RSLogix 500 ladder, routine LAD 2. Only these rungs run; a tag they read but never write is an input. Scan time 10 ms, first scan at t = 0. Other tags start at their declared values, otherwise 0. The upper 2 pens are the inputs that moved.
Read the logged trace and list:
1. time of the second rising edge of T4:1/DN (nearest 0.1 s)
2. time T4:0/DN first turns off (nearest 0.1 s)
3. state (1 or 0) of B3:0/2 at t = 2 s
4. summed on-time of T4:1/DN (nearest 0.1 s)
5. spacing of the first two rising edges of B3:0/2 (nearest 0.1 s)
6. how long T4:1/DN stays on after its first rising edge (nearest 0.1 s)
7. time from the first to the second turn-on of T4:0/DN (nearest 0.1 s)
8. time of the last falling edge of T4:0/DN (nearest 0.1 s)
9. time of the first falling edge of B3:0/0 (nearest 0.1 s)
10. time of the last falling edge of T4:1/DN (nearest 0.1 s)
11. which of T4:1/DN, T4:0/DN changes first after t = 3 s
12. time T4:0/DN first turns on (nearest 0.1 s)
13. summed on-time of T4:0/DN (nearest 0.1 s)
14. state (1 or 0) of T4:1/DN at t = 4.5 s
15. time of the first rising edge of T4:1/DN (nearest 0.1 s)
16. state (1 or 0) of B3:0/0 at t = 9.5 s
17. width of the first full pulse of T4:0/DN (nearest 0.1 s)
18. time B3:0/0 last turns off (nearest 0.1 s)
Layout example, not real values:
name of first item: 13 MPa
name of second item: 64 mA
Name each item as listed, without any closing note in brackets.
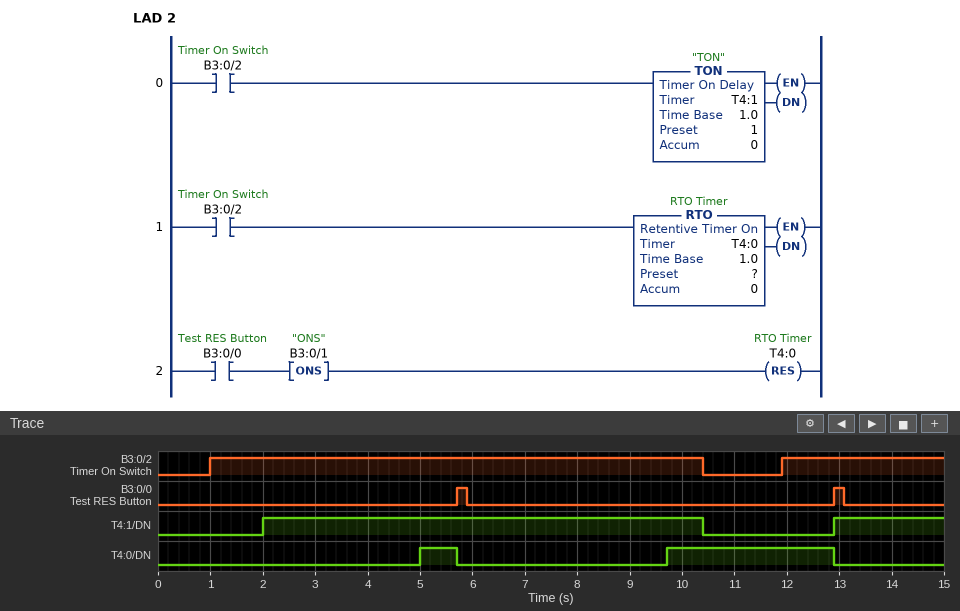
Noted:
time of the second rising edge of T4:1/DN: 12.9 s
time T4:0/DN first turns off: 5.7 s
state (1 or 0) of B3:0/2 at t = 2 s: 1
summed on-time of T4:1/DN: 10.5 s
spacing of the first two rising edges of B3:0/2: 10.9 s
how long T4:1/DN stays on after its first rising edge: 8.4 s
time from the first to the second turn-on of T4:0/DN: 4.7 s
time of the last falling edge of T4:0/DN: 12.9 s
time of the first falling edge of B3:0/0: 5.9 s
time of the last falling edge of T4:1/DN: 10.4 s
which of T4:1/DN, T4:0/DN changes first after t = 3 s: T4:0/DN
time T4:0/DN first turns on: 5.0 s
summed on-time of T4:0/DN: 3.9 s
state (1 or 0) of T4:1/DN at t = 4.5 s: 1
time of the first rising edge of T4:1/DN: 2.0 s
state (1 or 0) of B3:0/0 at t = 9.5 s: 0
width of the first full pulse of T4:0/DN: 0.7 s
time B3:0/0 last turns off: 13.1 s
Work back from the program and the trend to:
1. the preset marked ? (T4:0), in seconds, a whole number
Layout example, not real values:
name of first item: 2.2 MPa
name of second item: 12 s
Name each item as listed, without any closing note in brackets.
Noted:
the preset marked ? (T4:0), in seconds, a whole number: 4 s
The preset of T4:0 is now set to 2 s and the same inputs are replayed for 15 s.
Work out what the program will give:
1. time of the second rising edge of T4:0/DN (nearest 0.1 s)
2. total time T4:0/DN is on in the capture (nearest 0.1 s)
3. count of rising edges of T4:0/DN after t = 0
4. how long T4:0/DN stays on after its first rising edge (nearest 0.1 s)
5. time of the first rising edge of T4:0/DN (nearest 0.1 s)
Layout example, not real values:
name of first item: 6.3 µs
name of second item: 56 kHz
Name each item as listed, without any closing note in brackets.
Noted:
time of the second rising edge of T4:0/DN: 7.7 s
total time T4:0/DN is on in the capture: 8.0 s
count of rising edges of T4:0/DN after t = 0: 3
how long T4:0/DN stays on after its first rising edge: 2.7 s
time of the first rising edge of T4:0/DN: 3.0 s
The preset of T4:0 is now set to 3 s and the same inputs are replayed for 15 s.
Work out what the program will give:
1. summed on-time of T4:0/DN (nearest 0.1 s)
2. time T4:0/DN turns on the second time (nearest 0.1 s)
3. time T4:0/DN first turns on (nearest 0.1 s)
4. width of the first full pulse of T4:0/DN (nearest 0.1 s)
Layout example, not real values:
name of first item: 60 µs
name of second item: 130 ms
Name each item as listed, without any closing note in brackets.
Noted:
summed on-time of T4:0/DN: 5.9 s
time T4:0/DN turns on the second time: 8.7 s
time T4:0/DN first turns on: 4.0 s
width of the first full pulse of T4:0/DN: 1.7 s
